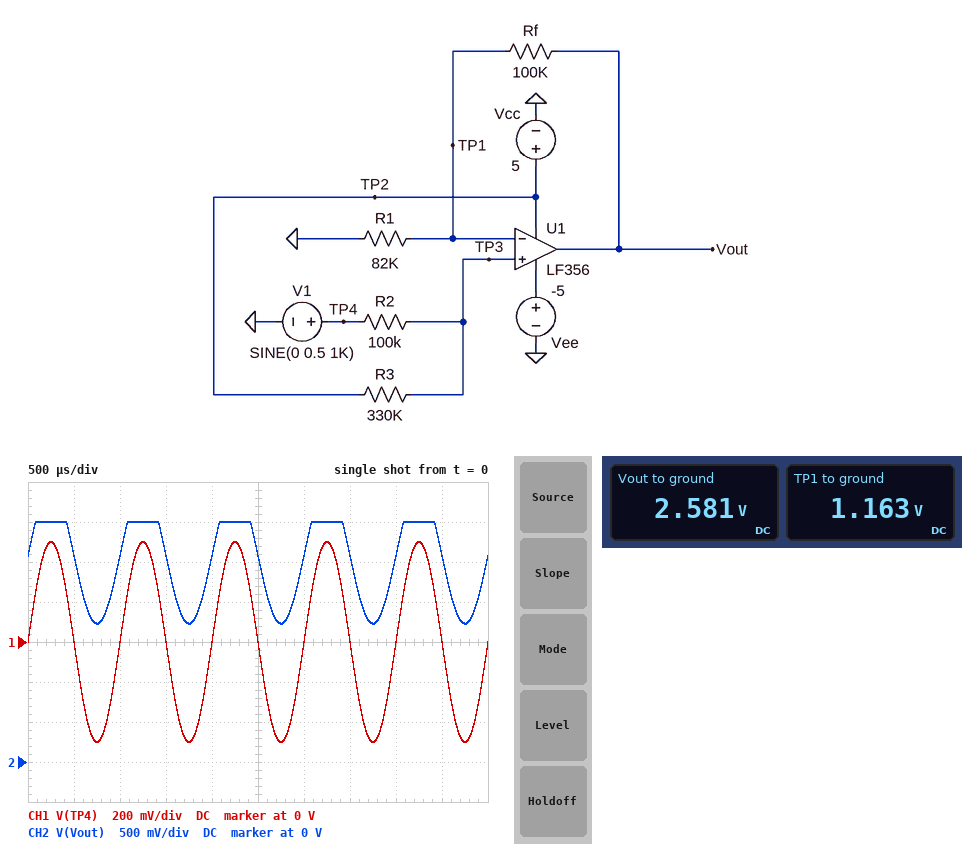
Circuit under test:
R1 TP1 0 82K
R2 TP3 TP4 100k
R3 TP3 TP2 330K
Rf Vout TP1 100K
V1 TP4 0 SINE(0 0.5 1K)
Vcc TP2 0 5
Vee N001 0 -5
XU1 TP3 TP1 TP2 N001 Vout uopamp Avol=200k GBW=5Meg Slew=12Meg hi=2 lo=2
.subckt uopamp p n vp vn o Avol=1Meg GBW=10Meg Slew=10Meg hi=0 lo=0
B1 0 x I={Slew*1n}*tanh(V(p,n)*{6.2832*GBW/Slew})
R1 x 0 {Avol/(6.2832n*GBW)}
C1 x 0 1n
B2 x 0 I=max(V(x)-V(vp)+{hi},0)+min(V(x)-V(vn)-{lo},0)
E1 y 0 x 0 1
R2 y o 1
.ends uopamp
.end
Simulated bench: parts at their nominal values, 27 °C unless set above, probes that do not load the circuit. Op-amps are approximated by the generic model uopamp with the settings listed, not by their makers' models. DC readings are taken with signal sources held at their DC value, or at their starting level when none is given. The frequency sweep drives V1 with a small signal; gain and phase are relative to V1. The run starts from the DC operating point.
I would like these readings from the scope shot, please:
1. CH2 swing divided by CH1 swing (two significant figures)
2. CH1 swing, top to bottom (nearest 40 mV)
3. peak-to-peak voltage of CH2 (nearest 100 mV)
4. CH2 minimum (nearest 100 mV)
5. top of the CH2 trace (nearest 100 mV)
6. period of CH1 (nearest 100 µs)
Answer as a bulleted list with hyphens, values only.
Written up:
- 1.3
- 1.00 V
- 1.3 V
- 1.7 V
- 3.0 V
- 1.0 ms
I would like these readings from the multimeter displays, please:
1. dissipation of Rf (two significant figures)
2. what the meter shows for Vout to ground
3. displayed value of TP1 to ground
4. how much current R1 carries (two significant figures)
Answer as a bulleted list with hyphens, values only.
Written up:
- 20 µW
- 2.581 V
- 1.163 V
- 14 µA
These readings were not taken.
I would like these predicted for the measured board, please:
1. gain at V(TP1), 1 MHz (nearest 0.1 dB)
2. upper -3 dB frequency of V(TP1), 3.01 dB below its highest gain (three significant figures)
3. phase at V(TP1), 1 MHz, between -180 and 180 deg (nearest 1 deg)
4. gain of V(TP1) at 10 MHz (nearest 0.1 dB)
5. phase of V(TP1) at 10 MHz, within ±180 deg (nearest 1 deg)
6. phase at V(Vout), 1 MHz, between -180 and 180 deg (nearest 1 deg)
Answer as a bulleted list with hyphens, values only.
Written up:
- -3.1 dB
- 2.25 MHz
- -24 deg
- -15.5 dB
- -77 deg
- -24 deg
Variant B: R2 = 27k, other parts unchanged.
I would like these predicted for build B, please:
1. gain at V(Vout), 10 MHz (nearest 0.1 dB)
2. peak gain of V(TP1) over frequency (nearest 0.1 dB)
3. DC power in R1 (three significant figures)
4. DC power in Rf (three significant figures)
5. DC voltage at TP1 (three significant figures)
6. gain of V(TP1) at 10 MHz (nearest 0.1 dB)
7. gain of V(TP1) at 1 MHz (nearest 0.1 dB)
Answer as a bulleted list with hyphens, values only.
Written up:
- -6.9 dB
- -0.7 dB
- 1.74 µW
- 2.13 µW
- 378 mV
- -13.8 dB
- -1.5 dB
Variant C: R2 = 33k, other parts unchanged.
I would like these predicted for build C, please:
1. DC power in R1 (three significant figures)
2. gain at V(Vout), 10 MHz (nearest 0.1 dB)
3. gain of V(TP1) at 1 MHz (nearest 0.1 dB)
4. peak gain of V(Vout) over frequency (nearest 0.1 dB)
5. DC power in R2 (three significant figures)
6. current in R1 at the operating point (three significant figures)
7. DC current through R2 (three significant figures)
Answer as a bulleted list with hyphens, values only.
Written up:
- 2.52 µW
- -7.1 dB
- -1.6 dB
- 6.1 dB
- 6.26 µW
- 5.54 µA
- 13.8 µA
